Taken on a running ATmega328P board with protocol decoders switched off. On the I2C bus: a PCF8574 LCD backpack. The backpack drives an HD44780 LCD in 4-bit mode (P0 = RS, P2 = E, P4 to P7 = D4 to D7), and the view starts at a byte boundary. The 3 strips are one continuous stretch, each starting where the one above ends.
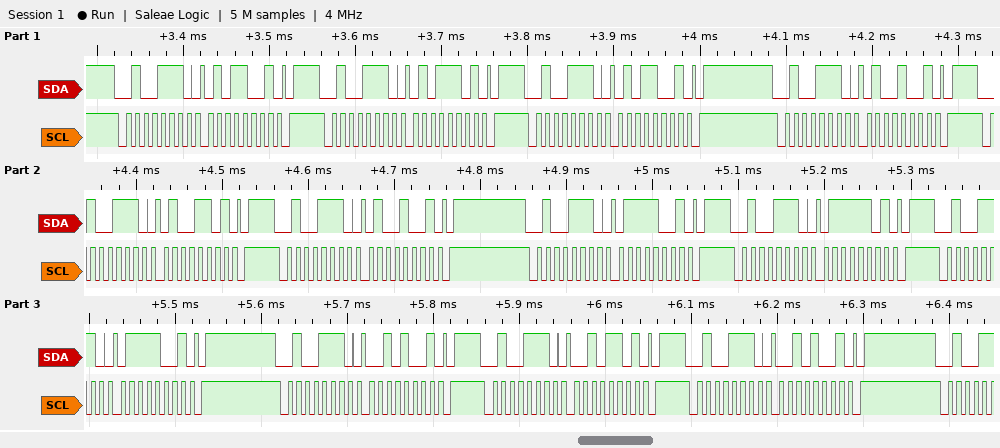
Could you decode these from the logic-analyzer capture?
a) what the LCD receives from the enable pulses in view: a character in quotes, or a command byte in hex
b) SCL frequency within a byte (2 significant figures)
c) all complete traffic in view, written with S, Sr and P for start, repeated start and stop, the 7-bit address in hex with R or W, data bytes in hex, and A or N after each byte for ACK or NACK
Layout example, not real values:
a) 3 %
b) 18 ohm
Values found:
a) 'T' 'r'
b) 100 kHz
c) S 27W A 59 A P S 27W A 5D A P S 27W A 59 A P S 27W A 49 A P S 27W A 4D A P S 27W A 49 A P S 27W A 79 A P S 27W A 7D A P S 27W A 79 A P S 27W A 29 A P S 27W A 2D A P S 27W A 29 A P
